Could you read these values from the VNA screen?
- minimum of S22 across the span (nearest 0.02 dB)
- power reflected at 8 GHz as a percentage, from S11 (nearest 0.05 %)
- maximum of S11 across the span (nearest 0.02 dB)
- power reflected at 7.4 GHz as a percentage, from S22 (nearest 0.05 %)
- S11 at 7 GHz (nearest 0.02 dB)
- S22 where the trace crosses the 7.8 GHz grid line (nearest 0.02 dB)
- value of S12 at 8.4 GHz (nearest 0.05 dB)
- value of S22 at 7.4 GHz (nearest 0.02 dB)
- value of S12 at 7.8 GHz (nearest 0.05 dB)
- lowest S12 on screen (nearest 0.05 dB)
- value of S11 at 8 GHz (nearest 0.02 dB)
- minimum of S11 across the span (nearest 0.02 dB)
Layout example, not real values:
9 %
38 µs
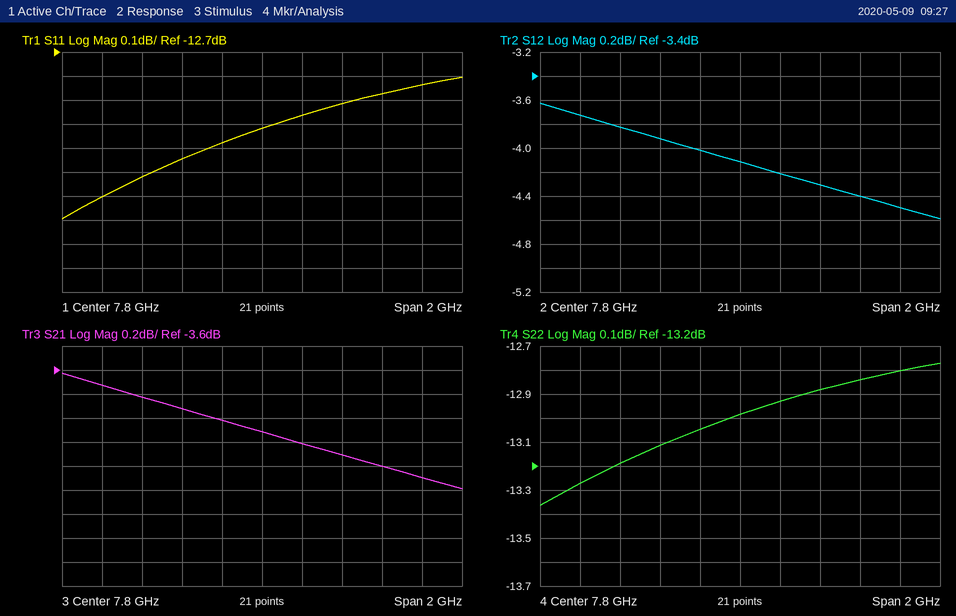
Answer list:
-13.36 dB
5.05 %
-12.80 dB
4.90 %
-13.30 dB
-12.98 dB
-4.40 dB
-13.12 dB
-4.10 dB
-4.60 dB
-12.96 dB
-13.40 dB
